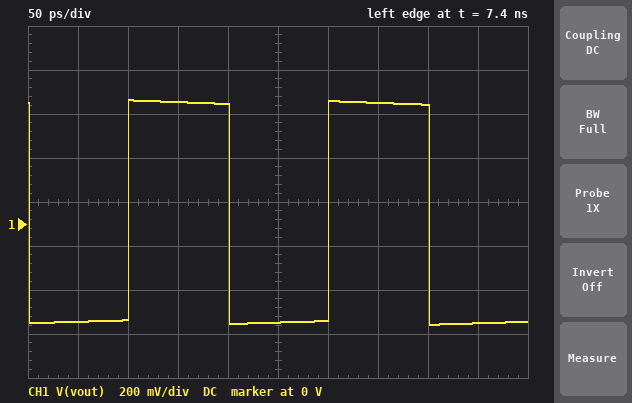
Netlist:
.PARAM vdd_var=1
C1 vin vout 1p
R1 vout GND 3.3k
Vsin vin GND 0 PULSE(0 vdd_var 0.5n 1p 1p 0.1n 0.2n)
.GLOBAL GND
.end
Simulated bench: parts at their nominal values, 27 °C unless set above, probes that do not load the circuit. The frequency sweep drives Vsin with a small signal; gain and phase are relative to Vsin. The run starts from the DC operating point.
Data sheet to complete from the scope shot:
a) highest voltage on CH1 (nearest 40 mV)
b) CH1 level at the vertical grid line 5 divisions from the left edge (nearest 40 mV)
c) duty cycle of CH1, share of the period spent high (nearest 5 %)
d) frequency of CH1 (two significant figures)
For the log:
560 mV
-440 mV
50 %
5.0 GHz
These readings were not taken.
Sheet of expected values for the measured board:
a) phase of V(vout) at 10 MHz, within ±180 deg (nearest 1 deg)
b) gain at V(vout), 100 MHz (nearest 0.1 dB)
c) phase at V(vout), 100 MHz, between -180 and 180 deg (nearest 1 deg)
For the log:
78 deg
-0.9 dB
26 deg
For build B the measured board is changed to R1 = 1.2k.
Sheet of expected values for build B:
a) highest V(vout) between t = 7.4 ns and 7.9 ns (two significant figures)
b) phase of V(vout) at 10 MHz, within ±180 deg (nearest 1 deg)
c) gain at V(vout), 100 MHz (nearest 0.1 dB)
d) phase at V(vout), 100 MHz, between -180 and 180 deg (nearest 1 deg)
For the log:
520 mV
86 deg
-4.4 dB
53 deg
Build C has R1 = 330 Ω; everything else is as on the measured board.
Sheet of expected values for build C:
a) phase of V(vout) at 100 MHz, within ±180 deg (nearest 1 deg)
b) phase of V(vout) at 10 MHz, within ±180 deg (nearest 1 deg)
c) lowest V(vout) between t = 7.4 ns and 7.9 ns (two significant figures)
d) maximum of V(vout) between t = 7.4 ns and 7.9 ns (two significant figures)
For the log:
78 deg
89 deg
-580 mV
570 mV
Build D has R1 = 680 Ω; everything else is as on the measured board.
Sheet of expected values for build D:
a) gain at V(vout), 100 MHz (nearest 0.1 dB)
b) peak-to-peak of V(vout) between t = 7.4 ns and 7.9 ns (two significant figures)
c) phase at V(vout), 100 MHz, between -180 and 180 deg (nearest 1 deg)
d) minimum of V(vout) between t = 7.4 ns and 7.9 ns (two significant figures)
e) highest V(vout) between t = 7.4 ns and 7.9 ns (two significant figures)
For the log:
-8.1 dB
1.1 V
67 deg
-540 mV
530 mV
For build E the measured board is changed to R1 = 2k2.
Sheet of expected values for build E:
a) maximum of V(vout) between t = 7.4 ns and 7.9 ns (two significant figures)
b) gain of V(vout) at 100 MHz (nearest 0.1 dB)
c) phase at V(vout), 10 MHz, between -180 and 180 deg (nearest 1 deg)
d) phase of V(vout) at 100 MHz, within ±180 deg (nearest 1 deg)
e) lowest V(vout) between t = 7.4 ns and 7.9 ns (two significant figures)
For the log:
530 mV
-1.8 dB
82 deg
36 deg
-500 mV
